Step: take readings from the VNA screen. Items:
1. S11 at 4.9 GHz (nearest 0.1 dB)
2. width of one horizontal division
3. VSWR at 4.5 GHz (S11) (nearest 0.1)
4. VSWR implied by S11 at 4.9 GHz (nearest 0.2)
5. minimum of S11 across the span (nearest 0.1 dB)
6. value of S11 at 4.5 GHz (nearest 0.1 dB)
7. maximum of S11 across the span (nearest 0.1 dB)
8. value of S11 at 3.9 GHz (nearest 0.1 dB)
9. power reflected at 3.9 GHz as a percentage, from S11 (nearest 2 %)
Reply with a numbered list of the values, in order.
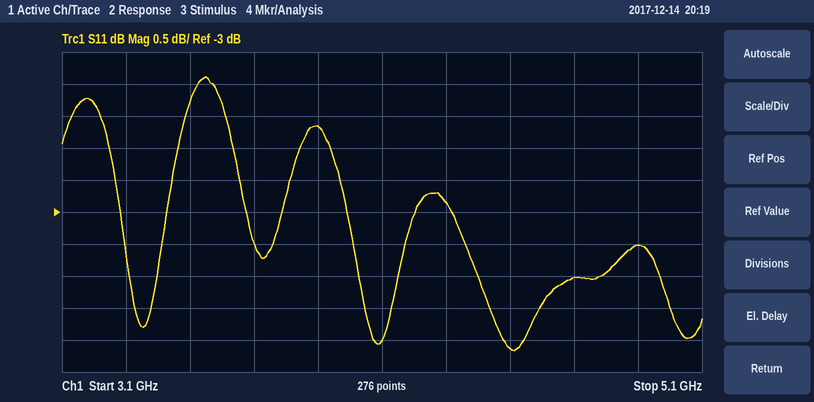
1. -3.5 dB
2. 200 MHz
3. 3.5
4. 5.0
5. -5.2 dB
6. -5.1 dB
7. -0.9 dB
8. -1.7 dB
9. 68 %
